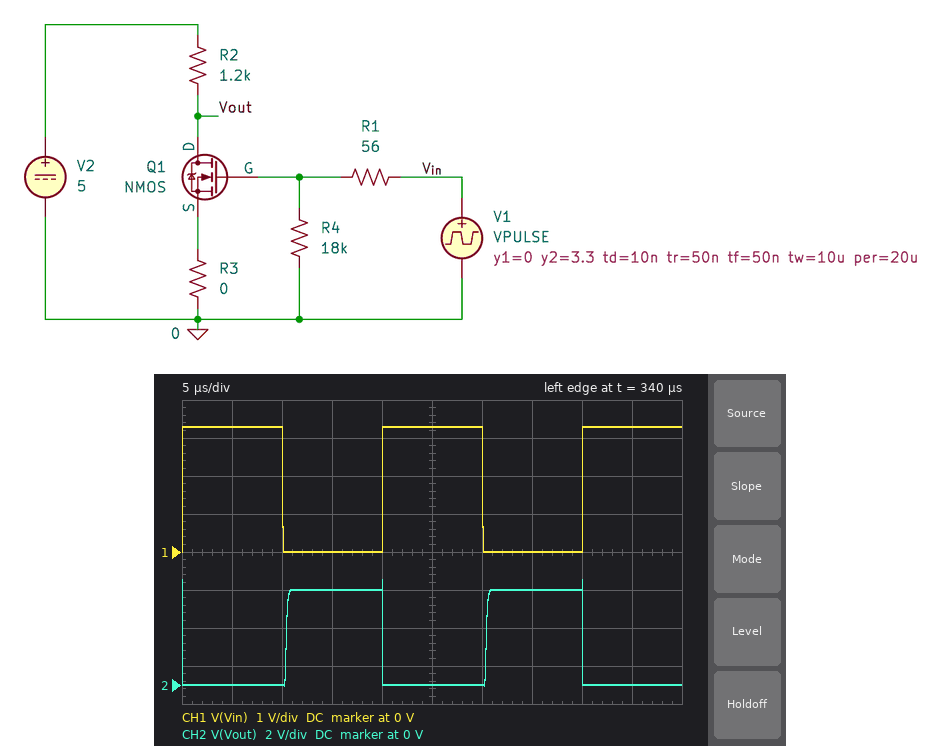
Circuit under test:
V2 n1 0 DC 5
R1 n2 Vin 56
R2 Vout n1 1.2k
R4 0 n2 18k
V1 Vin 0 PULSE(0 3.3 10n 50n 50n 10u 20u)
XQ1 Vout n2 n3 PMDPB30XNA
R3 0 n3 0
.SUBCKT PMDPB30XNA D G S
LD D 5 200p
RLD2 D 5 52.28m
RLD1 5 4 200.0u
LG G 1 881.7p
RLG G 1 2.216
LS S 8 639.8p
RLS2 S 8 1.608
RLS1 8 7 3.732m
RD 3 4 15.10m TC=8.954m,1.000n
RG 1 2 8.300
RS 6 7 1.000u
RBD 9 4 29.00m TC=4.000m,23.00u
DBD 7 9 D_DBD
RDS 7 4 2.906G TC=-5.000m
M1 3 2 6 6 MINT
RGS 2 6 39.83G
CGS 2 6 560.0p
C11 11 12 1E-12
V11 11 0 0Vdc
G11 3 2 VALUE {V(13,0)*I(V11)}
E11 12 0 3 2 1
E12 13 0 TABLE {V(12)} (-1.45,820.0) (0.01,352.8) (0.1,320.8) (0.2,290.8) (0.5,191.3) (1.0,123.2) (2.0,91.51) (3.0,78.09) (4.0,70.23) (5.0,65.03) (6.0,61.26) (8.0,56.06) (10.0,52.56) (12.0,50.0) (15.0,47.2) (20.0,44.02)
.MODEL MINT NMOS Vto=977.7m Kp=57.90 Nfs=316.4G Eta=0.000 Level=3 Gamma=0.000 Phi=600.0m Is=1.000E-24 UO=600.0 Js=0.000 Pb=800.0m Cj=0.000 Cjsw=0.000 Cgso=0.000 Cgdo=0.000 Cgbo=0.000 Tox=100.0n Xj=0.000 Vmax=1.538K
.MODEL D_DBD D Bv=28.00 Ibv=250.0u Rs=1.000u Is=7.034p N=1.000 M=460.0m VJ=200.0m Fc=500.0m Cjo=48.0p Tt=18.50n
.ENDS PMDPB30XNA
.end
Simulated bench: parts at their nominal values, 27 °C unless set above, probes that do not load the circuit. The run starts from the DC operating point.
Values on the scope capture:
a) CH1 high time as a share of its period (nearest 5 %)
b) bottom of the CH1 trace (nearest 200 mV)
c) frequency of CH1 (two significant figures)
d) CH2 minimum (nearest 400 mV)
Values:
50 %
0 V
50 kHz
0 V
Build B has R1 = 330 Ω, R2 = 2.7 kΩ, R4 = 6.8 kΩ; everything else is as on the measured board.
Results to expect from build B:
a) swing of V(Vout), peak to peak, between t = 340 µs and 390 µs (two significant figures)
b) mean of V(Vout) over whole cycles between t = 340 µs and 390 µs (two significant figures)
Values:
5.5 V
2.2 V
